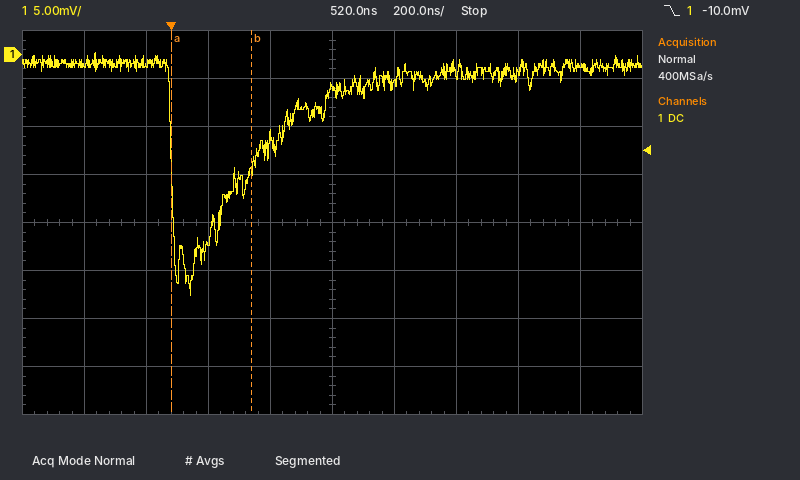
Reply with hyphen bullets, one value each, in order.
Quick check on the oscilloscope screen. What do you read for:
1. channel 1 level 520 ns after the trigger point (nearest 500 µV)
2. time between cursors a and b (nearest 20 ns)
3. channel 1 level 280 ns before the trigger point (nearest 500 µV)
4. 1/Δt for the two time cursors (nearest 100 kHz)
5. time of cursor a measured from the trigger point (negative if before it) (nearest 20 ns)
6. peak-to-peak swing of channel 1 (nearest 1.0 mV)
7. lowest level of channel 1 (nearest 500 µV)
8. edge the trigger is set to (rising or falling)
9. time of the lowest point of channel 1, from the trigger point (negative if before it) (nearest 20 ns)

- -3.5 mV
- 260 ns
- -1.0 mV
- 3.8 MHz
- 0 ns
- 25.0 mV
- -25.0 mV
- falling
- +60 ns
